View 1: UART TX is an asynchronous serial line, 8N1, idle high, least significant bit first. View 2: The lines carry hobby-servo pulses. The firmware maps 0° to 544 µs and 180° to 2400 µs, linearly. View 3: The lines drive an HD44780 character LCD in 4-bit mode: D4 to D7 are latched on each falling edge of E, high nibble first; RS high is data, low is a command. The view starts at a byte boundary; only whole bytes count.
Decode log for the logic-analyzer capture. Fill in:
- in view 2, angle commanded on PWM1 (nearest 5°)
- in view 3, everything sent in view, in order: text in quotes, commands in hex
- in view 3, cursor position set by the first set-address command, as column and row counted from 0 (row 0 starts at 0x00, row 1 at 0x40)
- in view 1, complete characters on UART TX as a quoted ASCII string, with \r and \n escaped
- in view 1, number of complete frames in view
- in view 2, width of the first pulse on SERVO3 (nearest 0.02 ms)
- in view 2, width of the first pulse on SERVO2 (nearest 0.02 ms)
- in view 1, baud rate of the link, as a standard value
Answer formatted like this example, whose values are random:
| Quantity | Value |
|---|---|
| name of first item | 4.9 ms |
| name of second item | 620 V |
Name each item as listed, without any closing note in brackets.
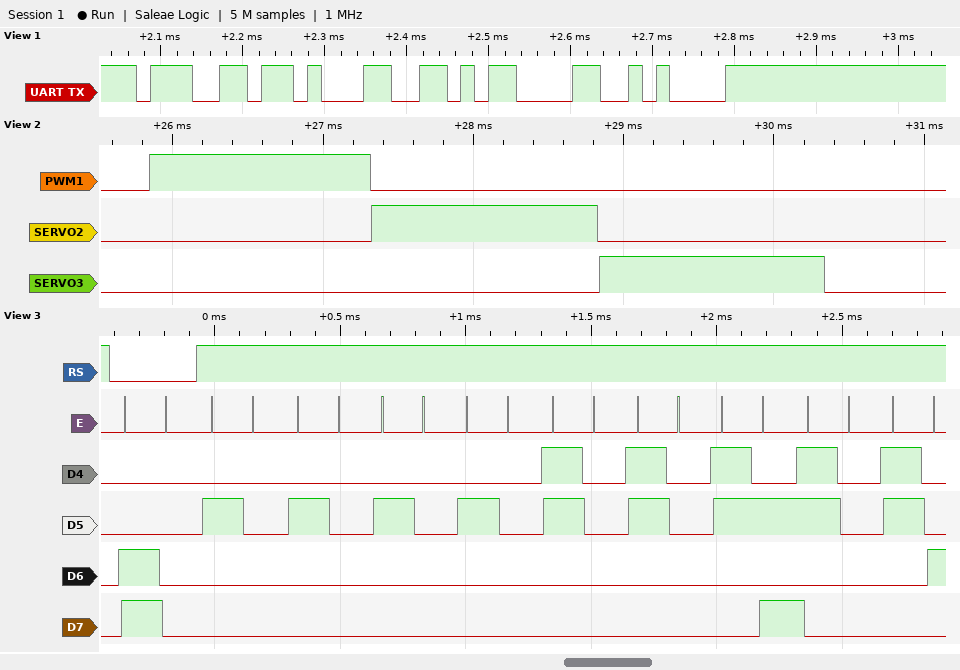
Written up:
| Quantity | Value |
|---|---|
| in view 2, angle commanded on PWM1 | 90° |
| in view 3, everything sent in view, in order: text in quotes, commands in hex | 0xC0 "    00:04" |
| in view 3, cursor position set by the first set-address command, as column and row counted from 0 | column 0, row 1 |
| in view 1, complete characters on UART TX as a quoted ASCII string, with \r and \n escaped | "g1\r\n" |
| in view 1, number of complete frames in view | 4 |
| in view 2, width of the first pulse on SERVO3 | 1.50 ms |
| in view 2, width of the first pulse on SERVO2 | 1.50 ms |
| in view 1, baud rate of the link, as a standard value | 57600 baud |
